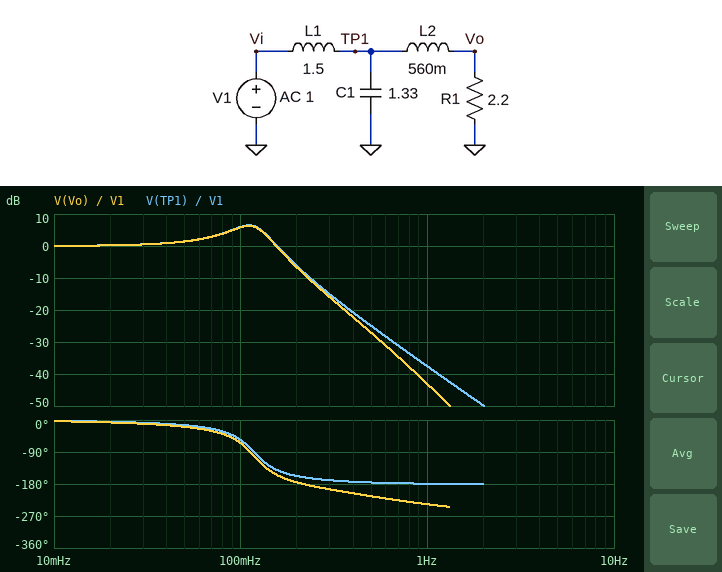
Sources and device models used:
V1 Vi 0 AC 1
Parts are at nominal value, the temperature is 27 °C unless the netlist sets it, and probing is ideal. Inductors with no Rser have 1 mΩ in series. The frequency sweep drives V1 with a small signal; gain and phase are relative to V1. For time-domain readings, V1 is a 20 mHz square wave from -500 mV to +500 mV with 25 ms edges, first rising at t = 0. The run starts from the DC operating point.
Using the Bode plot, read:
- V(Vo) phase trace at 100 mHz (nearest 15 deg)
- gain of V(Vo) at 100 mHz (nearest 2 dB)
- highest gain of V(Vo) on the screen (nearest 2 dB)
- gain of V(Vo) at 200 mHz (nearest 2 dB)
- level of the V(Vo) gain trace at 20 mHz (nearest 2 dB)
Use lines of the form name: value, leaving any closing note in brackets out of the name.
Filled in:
V(Vo) phase trace at 100 mHz: -60 deg
gain of V(Vo) at 100 mHz: 6 dB
highest gain of V(Vo) on the screen: 6 dB
gain of V(Vo) at 200 mHz: -6 dB
level of the V(Vo) gain trace at 20 mHz: 0 dB
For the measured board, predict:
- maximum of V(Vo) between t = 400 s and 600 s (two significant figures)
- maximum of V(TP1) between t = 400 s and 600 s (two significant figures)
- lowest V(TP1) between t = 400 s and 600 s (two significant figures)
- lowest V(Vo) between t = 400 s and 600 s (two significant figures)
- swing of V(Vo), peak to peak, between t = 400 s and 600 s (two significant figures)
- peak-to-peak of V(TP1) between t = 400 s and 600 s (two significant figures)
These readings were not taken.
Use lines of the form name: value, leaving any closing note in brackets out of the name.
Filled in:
maximum of V(Vo) between t = 400 s and 600 s: 940 mV
maximum of V(TP1) between t = 400 s and 600 s: 950 mV
lowest V(TP1) between t = 400 s and 600 s: -950 mV
lowest V(Vo) between t = 400 s and 600 s: -940 mV
swing of V(Vo), peak to peak, between t = 400 s and 600 s: 1.9 V
peak-to-peak of V(TP1) between t = 400 s and 600 s: 1.9 V
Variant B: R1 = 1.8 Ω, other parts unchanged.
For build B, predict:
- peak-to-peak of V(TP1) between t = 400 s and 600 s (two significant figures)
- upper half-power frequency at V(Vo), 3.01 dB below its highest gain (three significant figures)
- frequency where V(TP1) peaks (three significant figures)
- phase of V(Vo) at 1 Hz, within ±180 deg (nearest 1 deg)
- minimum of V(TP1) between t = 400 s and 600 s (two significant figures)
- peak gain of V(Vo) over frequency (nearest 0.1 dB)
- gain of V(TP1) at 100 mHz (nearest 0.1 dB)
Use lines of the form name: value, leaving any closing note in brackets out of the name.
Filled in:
peak-to-peak of V(TP1) between t = 400 s and 600 s: 1.7 V
upper half-power frequency at V(Vo), 3.01 dB below its highest gain: 142 mHz
frequency where V(TP1) peaks: 110 mHz
phase of V(Vo) at 1 Hz, within ±180 deg: 118 deg
minimum of V(TP1) between t = 400 s and 600 s: -870 mV
peak gain of V(Vo) over frequency: 4.6 dB
gain of V(TP1) at 100 mHz: 4.5 dB
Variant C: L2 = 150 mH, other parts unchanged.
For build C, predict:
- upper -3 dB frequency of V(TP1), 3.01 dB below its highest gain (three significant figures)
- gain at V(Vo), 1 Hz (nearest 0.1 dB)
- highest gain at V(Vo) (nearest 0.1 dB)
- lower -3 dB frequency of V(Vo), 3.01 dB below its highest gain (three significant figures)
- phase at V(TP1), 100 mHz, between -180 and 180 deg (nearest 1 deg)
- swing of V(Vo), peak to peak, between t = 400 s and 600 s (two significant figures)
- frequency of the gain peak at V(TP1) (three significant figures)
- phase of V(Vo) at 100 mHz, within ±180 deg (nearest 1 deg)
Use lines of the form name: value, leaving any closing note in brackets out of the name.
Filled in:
upper -3 dB frequency of V(TP1), 3.01 dB below its highest gain: 133 mHz
gain at V(Vo), 1 Hz: -38.4 dB
highest gain at V(Vo): 6.5 dB
lower -3 dB frequency of V(Vo), 3.01 dB below its highest gain: 72.8 mHz
phase at V(TP1), 100 mHz, between -180 and 180 deg: -62 deg
swing of V(Vo), peak to peak, between t = 400 s and 600 s: 1.9 V
frequency of the gain peak at V(TP1): 107 mHz
phase of V(Vo) at 100 mHz, within ±180 deg: -64 deg
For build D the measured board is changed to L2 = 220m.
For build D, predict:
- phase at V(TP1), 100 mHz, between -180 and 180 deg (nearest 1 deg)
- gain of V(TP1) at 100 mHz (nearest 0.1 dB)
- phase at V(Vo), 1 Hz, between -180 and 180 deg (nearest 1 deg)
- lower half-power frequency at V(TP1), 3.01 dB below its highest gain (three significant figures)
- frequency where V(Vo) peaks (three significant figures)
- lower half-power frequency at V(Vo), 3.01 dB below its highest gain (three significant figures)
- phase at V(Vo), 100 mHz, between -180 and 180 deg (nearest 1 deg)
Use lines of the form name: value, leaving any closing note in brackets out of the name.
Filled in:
phase at V(TP1), 100 mHz, between -180 and 180 deg: -61 deg
gain of V(TP1) at 100 mHz: 6.2 dB
phase at V(Vo), 1 Hz, between -180 and 180 deg: 150 deg
lower half-power frequency at V(TP1), 3.01 dB below its highest gain: 73.1 mHz
frequency where V(Vo) peaks: 108 mHz
lower half-power frequency at V(Vo), 3.01 dB below its highest gain: 73.0 mHz
phase at V(Vo), 100 mHz, between -180 and 180 deg: -64 deg
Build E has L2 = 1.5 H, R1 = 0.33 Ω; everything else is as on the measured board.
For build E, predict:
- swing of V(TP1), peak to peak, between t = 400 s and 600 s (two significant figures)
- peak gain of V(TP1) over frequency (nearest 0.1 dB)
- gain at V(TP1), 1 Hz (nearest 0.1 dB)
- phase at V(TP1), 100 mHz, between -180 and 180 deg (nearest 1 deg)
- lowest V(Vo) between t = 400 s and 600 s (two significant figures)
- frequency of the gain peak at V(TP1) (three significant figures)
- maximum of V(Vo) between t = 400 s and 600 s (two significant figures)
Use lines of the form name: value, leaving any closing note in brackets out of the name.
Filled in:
swing of V(TP1), peak to peak, between t = 400 s and 600 s: 1.2 V
peak gain of V(TP1) over frequency: 13.4 dB
gain at V(TP1), 1 Hz: -37.7 dB
phase at V(TP1), 100 mHz, between -180 and 180 deg: -16 deg
lowest V(Vo) between t = 400 s and 600 s: -460 mV
frequency of the gain peak at V(TP1): 158 mHz
maximum of V(Vo) between t = 400 s and 600 s: 460 mV
